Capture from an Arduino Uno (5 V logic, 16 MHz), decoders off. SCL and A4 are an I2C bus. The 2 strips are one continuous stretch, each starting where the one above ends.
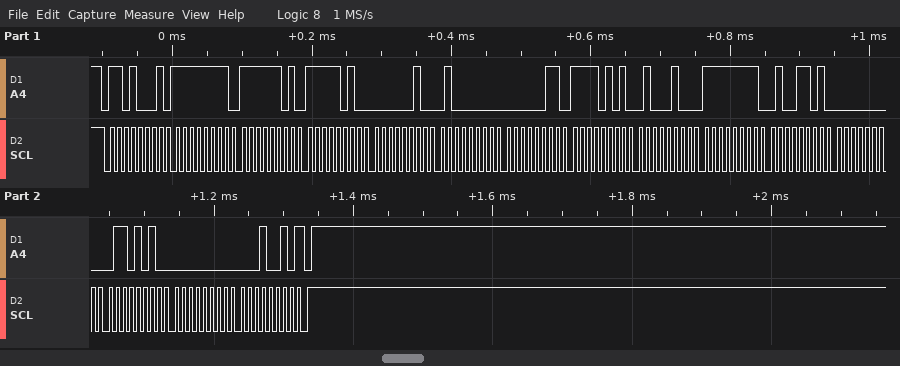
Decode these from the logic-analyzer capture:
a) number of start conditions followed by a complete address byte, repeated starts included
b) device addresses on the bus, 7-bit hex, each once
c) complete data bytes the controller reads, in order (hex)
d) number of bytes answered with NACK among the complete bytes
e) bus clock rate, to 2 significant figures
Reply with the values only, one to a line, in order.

1
0x68
FF FD FA 02 40 03 F5 44 FF 4D 00 6A 00 12
1
100 kHz
